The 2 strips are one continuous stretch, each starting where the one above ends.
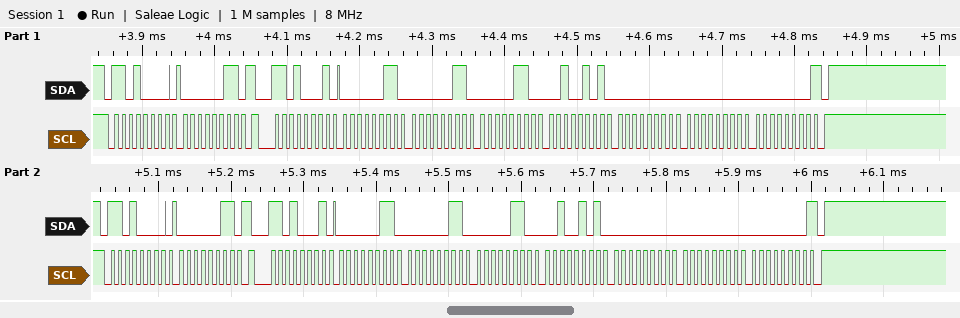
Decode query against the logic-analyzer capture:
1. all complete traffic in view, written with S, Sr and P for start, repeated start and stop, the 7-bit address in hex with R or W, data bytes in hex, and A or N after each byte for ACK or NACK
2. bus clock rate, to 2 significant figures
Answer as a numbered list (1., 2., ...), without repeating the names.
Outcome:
1. S 68W A 03 A Sr 68R A 03 A 03 A 06 A 25 A 00 A 00 A 00 N P S 68W A 03 A Sr 68R A 03 A 03 A 06 A 25 A 00 A 00 A 00 N P
2. 100 kHz
